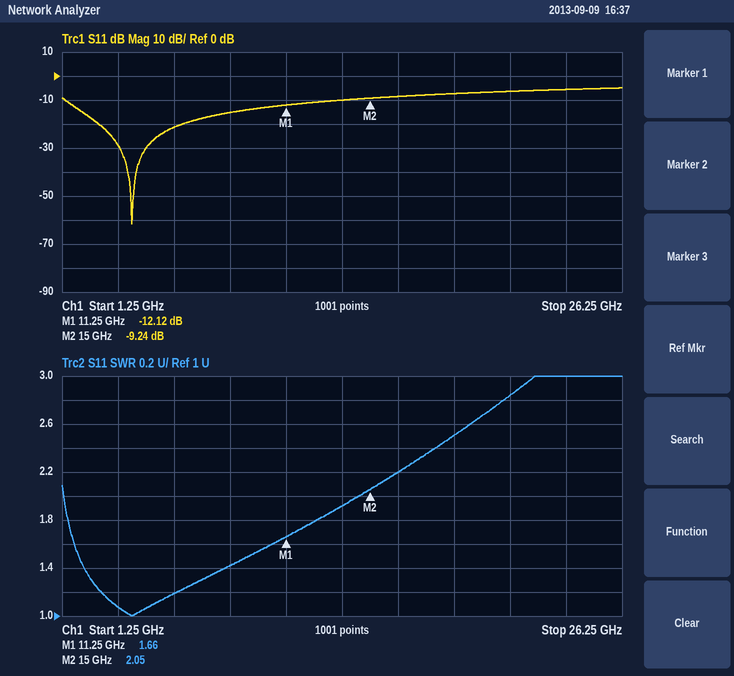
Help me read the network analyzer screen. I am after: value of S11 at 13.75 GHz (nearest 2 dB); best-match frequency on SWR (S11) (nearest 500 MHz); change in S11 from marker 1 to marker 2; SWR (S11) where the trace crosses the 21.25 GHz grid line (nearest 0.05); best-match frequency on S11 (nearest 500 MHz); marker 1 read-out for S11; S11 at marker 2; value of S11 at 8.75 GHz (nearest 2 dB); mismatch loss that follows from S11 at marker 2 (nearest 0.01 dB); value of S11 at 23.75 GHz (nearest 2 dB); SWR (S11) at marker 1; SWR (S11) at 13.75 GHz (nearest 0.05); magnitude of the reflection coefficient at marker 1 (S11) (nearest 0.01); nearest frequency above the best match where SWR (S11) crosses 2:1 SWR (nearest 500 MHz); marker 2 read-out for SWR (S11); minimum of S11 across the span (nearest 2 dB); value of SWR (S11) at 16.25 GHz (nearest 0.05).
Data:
-10 dB
4.5 GHz
2.88 dB
2.85
4.5 GHz
-12.12 dB
-9.24 dB
-16 dB
0.55 dB
-6 dB
1.66
1.90
0.25
14.5 GHz
2.05
-62 dB
2.20
